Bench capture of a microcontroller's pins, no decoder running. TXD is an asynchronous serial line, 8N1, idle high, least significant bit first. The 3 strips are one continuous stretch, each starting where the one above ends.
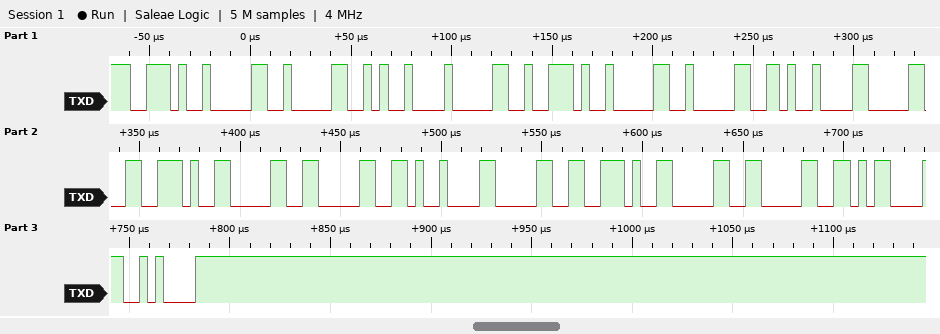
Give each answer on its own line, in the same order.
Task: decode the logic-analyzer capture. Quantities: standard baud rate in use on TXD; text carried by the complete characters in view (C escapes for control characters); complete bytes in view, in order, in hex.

250000 baud
".00\t0.00\t0.00\t0.00\r\n"
2E 30 30 09 30 2E 30 30 09 30 2E 30 30 09 30 2E 30 30 0D 0A
